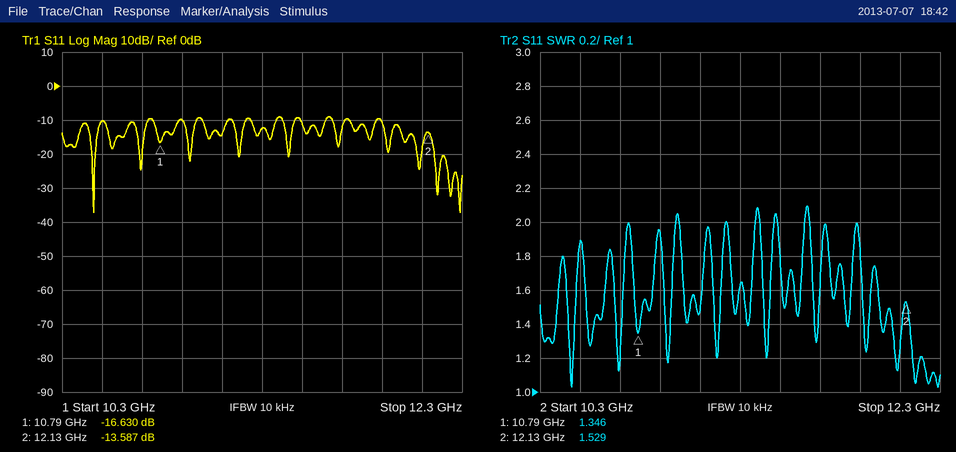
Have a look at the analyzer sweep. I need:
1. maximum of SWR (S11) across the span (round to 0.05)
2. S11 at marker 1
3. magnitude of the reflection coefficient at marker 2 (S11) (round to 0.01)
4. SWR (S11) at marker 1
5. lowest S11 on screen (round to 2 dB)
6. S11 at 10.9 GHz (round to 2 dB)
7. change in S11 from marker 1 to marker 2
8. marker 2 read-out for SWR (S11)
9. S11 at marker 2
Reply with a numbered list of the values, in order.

1. 2.10
2. -16.630 dB
3. 0.21
4. 1.346
5. -38 dB
6. -10 dB
7. 3.043 dB
8. 1.529
9. -13.587 dB
